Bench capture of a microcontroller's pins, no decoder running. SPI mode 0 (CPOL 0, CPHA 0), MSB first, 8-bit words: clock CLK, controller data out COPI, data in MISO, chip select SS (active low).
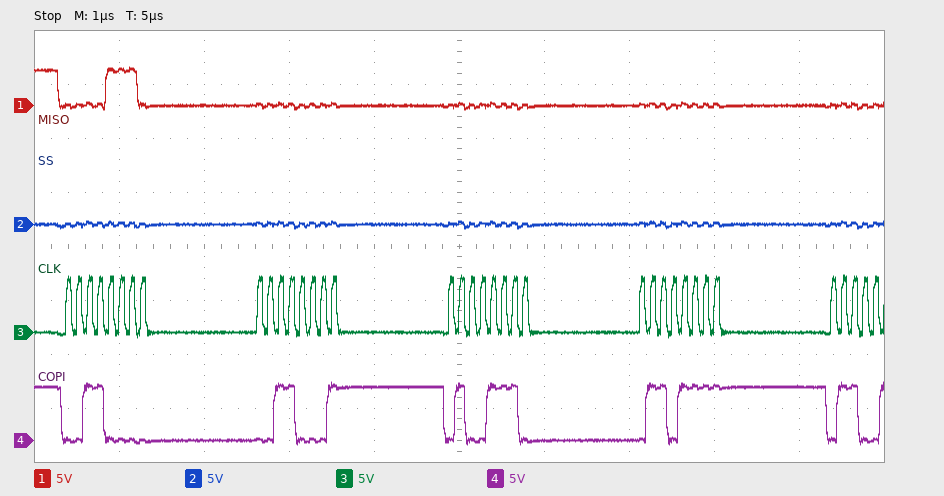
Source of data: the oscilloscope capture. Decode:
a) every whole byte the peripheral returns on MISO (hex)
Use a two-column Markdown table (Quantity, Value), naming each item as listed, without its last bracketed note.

| Quantity | Value |
|---|---|
| every whole byte the peripheral returns on MISO | 0E 00 00 00 |
